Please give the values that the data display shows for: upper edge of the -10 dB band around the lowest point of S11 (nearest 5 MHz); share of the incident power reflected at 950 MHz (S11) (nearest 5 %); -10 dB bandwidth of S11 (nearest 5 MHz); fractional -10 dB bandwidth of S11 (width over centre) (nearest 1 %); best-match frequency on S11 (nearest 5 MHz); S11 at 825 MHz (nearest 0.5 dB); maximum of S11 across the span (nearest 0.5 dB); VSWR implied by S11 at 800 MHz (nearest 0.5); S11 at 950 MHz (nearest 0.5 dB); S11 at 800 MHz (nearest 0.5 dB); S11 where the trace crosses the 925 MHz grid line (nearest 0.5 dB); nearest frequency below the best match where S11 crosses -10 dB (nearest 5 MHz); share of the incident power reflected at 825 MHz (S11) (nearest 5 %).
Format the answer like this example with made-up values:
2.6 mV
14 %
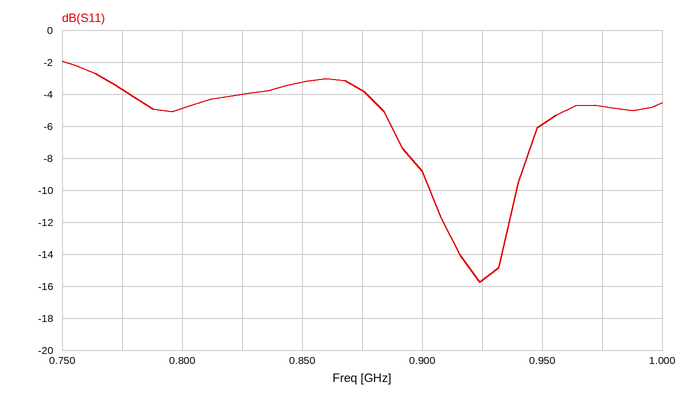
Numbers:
940 MHz
25 %
35 MHz
4 %
925 MHz
-4.0 dB
-2.0 dB
3.5
-6.0 dB
-5.0 dB
-15.5 dB
905 MHz
40 %
